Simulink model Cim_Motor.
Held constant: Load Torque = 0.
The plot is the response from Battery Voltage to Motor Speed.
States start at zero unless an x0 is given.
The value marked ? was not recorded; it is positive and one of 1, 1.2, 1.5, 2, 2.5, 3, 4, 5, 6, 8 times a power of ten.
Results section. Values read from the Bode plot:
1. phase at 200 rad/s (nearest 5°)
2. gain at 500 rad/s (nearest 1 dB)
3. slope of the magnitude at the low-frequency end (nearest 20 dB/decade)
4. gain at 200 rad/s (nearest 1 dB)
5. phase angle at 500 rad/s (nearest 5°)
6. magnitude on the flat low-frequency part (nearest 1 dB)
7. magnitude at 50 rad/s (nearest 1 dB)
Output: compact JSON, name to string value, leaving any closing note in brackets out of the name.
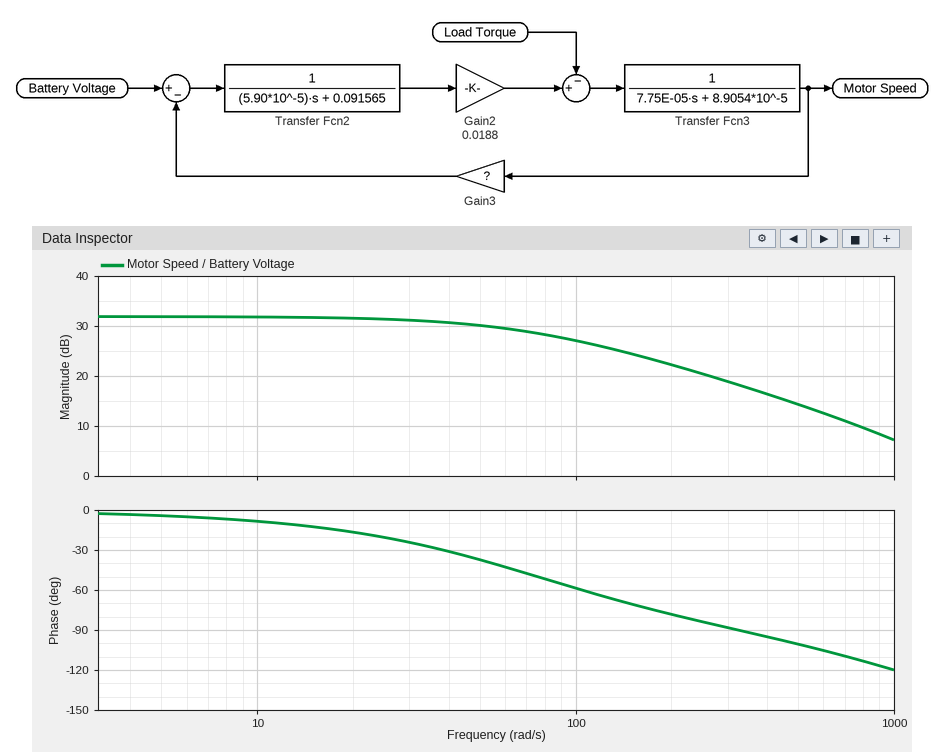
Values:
{"phase at 200 rad/s": "-80°", "gain at 500 rad/s": "14 dB", "slope of the magnitude at the low-frequency end": "0 dB/decade", "gain at 200 rad/s": "22 dB", "phase angle at 500 rad/s": "-100°", "magnitude on the flat low-frequency part": "32 dB", "magnitude at 50 rad/s": "30 dB"}
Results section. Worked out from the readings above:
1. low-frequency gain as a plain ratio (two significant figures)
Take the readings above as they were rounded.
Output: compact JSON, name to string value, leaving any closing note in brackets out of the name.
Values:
{"low-frequency gain as a plain ratio": "40"}
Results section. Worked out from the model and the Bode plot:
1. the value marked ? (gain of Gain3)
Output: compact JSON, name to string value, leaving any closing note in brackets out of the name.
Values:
{"the value marked ?": "0.025"}
